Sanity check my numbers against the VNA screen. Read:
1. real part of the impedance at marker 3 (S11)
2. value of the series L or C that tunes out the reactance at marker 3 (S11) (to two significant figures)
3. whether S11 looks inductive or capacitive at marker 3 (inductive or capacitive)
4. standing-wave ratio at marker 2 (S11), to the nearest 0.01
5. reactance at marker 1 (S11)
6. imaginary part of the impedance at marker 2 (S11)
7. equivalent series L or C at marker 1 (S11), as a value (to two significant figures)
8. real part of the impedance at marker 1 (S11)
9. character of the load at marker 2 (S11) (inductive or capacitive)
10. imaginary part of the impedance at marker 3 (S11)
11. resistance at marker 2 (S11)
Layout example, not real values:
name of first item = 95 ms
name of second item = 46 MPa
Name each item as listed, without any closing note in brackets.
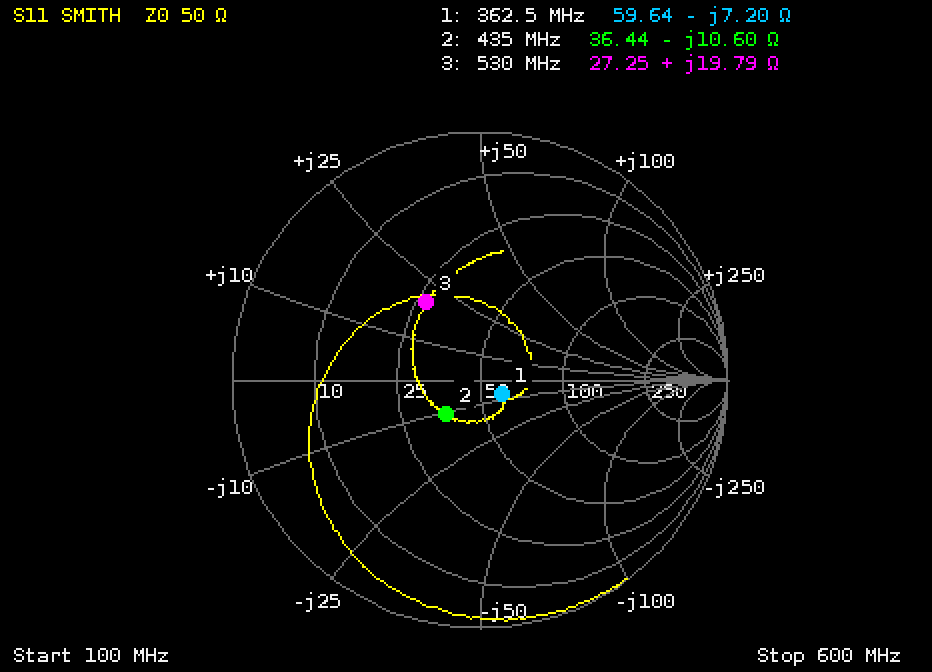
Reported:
real part of the impedance at marker 3 = 27.25 Ω
value of the series L or C that tunes out the reactance at marker 3 (S11) = 15 pF
whether S11 looks inductive or capacitive at marker 3 = inductive
standing-wave ratio at marker 2 (S11), to the nearest 0.01 = 1.49
reactance at marker 1 = -7.20 Ω
imaginary part of the impedance at marker 2 = -10.60 Ω
equivalent series L or C at marker 1 (S11), as a value = 61 pF
real part of the impedance at marker 1 = 59.64 Ω
character of the load at marker 2 (S11) = capacitive
imaginary part of the impedance at marker 3 = +19.79 Ω
resistance at marker 2 = 36.44 Ω
